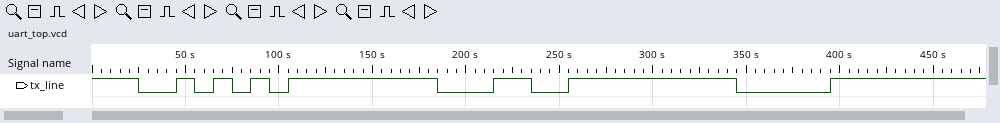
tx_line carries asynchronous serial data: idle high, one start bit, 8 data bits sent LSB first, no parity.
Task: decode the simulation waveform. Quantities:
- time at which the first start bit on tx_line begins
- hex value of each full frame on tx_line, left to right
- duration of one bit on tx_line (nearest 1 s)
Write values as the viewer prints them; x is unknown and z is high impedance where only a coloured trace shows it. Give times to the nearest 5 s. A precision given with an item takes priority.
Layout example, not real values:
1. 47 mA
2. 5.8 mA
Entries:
1. 25 s
2. AA, CC, F0
3. 10 s
